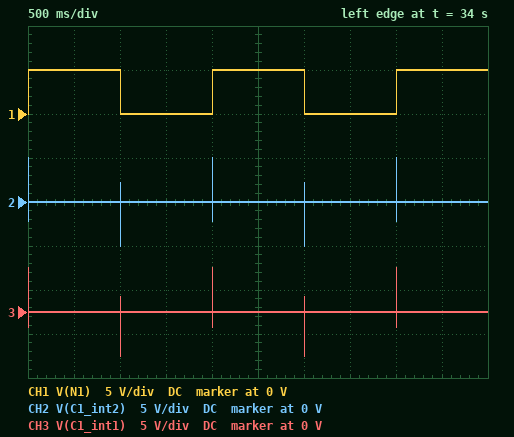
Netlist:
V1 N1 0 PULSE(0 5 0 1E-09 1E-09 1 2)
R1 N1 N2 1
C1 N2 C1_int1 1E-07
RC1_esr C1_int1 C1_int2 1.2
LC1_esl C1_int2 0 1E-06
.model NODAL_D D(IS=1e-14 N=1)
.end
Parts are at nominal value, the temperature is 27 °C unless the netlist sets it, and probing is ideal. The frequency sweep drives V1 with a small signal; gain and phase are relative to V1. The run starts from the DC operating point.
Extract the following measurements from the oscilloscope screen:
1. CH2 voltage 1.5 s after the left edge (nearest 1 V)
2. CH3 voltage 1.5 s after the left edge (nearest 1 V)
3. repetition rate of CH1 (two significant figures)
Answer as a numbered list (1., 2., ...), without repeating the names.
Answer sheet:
1. 0 V
2. 0 V
3. 500 mHz
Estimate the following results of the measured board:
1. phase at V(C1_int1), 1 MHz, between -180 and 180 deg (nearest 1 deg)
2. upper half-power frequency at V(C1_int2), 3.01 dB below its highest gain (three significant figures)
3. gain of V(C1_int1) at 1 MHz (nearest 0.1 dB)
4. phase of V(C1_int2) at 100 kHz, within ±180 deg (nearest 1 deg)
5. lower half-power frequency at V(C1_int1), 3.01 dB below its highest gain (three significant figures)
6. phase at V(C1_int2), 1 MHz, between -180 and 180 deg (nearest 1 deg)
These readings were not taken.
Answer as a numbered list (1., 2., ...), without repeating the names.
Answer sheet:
1. 14 deg
2. 1.55 MHz
3. 1.8 dB
4. 172 deg
5. 416 kHz
6. 25 deg
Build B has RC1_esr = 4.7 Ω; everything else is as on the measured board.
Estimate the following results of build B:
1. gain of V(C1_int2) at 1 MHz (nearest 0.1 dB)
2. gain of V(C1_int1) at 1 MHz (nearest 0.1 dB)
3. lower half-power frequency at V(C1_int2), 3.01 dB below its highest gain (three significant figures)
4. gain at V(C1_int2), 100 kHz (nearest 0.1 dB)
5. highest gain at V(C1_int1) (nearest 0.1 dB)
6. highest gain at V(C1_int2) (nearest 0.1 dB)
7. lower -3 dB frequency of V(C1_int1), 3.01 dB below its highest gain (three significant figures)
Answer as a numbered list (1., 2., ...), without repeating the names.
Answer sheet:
1. -1.4 dB
2. 0.5 dB
3. 676 kHz
4. -28.3 dB
5. 0.6 dB
6. 0 dB
7. 296 kHz
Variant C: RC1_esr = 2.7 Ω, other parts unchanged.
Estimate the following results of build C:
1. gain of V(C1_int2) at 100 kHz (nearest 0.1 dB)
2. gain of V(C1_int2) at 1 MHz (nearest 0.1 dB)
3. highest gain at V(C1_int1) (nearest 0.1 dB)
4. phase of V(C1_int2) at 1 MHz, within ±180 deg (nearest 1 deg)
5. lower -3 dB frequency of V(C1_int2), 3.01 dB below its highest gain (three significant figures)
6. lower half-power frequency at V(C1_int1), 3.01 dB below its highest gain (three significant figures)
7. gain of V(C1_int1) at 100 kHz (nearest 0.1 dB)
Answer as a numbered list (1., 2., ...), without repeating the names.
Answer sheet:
1. -28.0 dB
2. 0.4 dB
3. 1.7 dB
4. 38 deg
5. 448 kHz
6. 373 kHz
7. -15.1 dB
